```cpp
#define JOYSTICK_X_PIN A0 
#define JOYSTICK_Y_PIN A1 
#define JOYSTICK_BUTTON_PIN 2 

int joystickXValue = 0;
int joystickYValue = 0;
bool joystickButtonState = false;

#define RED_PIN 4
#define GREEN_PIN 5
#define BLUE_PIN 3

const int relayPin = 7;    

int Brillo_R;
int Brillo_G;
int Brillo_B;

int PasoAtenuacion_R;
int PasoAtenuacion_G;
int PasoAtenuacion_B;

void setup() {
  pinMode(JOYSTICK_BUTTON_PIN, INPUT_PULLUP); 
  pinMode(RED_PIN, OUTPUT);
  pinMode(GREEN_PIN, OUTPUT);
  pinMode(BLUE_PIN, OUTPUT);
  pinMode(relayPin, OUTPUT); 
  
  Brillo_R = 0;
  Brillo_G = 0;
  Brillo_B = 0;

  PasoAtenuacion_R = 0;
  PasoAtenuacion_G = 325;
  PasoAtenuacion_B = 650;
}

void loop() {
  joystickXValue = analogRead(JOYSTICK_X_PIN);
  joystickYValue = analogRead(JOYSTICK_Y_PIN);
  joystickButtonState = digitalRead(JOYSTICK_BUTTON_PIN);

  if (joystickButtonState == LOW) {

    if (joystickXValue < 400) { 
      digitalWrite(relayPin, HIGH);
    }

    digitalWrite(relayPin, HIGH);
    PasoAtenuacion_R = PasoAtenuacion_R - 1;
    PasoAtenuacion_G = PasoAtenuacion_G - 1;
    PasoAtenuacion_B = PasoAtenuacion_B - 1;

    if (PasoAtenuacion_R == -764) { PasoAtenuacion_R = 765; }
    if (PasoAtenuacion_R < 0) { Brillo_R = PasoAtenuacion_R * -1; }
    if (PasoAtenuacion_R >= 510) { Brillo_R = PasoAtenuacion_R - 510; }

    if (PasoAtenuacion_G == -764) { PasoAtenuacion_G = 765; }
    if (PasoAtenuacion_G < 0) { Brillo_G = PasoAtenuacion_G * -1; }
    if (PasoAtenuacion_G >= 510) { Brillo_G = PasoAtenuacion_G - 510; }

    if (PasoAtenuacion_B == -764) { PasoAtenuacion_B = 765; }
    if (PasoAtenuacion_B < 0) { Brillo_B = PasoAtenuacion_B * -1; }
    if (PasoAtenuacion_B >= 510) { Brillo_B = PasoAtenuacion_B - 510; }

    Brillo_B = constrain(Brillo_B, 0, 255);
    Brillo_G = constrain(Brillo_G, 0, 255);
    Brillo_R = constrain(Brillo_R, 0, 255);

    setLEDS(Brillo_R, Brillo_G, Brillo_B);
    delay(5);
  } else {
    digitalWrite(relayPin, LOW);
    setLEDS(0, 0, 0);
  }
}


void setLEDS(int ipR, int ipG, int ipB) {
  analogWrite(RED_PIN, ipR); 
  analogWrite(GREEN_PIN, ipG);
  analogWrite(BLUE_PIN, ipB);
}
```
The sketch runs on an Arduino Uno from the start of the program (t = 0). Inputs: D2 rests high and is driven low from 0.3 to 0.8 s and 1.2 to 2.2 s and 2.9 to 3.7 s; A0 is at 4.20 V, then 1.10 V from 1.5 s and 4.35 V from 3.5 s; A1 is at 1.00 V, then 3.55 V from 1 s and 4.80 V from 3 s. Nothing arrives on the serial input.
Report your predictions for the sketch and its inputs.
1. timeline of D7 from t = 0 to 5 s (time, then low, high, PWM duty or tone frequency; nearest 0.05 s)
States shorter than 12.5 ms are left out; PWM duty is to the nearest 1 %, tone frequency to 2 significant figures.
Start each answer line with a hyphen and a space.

- 0 s low; 0.3 s high; 0.8 s low; 1.2 s high; 2.2 s low; 2.9 s high; 3.7 s low
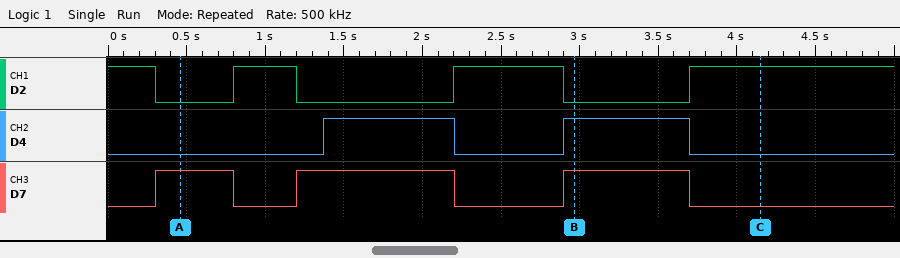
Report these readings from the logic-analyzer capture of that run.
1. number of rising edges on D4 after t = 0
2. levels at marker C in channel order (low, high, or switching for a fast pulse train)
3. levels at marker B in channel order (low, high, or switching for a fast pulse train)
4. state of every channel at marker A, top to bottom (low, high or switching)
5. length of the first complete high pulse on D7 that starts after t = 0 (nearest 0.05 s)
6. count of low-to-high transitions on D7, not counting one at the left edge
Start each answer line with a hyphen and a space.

- 2
- D2 high, D4 low, D7 low
- D2 low, D4 high, D7 high
- D2 low, D4 low, D7 high
- 0.50 s
- 3
